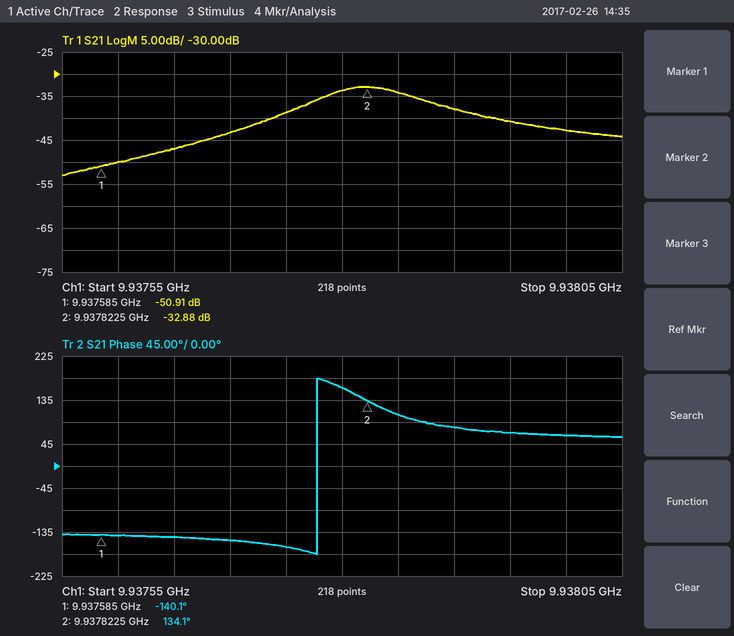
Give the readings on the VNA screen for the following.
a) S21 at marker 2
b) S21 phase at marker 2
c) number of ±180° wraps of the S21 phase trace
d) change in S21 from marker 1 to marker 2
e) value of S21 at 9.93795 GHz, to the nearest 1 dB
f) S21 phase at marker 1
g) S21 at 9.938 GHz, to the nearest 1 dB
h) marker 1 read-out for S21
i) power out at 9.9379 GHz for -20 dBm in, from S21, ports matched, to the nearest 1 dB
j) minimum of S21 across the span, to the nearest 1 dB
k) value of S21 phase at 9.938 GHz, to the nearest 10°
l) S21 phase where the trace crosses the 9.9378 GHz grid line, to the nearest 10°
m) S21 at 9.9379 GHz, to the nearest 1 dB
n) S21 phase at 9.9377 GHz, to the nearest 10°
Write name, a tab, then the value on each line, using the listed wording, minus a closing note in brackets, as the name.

S21 at marker 2	-32.88 dB
S21 phase at marker 2	134.1°
number of ±180° wraps of the S21 phase trace	1
change in S21 from marker 1 to marker 2	18.03 dB
value of S21 at 9.93795 GHz, to the nearest 1 dB	-41 dB
S21 phase at marker 1	-140.1°
S21 at 9.938 GHz, to the nearest 1 dB	-43 dB
marker 1 read-out for S21	-50.91 dB
power out at 9.9379 GHz for -20 dBm in, from S21, ports matched, to the nearest 1 dB	-58 dBm
minimum of S21 across the span, to the nearest 1 dB	-53 dB
value of S21 phase at 9.938 GHz, to the nearest 10°	60°
S21 phase where the trace crosses the 9.9378 GHz grid line, to the nearest 10°	160°
S21 at 9.9379 GHz, to the nearest 1 dB	-38 dB
S21 phase at 9.9377 GHz, to the nearest 10°	-150°
